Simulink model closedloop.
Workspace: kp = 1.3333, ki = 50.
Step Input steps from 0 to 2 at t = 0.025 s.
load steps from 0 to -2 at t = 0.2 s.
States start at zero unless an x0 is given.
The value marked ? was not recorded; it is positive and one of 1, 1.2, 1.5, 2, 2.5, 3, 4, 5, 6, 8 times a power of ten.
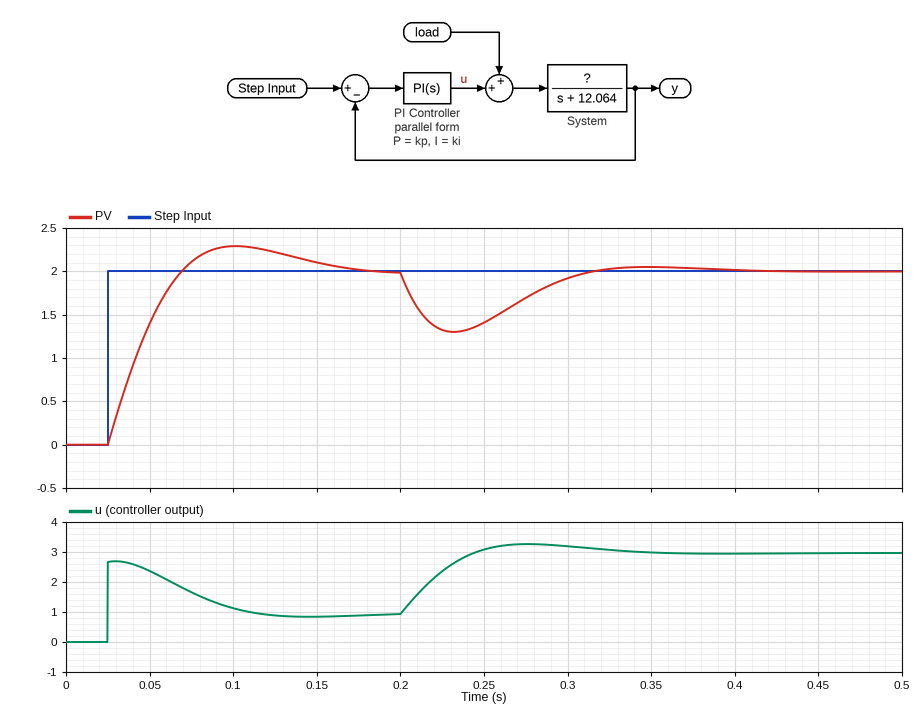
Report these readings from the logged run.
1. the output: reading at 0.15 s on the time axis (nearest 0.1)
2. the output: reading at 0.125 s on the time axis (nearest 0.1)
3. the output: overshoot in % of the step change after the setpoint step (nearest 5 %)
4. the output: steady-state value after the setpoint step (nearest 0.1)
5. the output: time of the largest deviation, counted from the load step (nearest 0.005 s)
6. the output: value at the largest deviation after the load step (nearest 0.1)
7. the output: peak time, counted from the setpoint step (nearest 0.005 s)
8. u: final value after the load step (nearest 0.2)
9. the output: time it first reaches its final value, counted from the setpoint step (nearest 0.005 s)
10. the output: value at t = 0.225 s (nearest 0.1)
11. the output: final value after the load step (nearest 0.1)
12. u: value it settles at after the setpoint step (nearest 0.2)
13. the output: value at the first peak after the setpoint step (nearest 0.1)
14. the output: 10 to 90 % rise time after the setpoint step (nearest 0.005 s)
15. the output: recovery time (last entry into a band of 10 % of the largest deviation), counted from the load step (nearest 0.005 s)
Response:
2.1
2.2
15 %
2.0
0.030 s
1.3
0.075 s
3.0
0.045 s
1.3
2.0
1.0
2.3
0.035 s
0.100 s
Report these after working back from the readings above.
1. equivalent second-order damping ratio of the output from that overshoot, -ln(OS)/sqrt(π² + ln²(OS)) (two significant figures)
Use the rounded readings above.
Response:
0.52
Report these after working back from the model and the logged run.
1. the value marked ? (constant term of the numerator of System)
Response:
25
